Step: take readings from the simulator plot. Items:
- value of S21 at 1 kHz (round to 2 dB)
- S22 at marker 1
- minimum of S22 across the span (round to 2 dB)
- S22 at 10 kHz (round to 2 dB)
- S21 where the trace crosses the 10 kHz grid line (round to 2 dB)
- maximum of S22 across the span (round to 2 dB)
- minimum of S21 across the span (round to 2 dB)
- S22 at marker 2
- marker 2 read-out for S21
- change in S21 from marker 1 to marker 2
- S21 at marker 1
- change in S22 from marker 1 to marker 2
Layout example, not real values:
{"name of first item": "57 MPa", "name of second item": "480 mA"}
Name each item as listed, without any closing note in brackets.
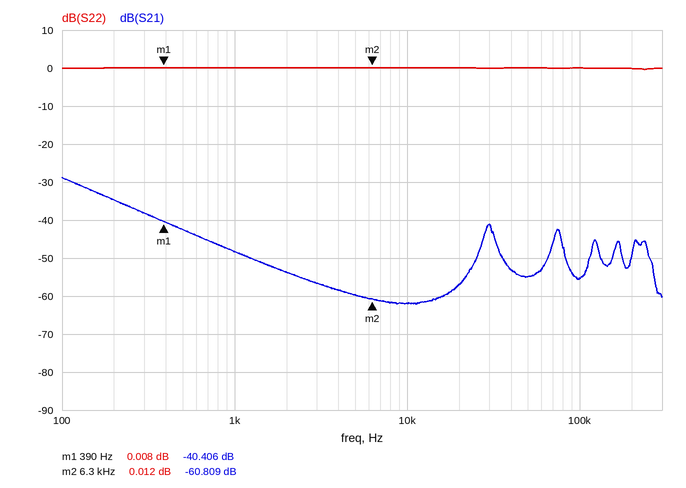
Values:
{"value of S21 at 1 kHz": "-48 dB", "S22 at marker 1": "0.008 dB", "minimum of S22 across the span": "0 dB", "S22 at 10 kHz": "0 dB", "S21 where the trace crosses the 10 kHz grid line": "-62 dB", "maximum of S22 across the span": "0 dB", "minimum of S21 across the span": "-62 dB", "S22 at marker 2": "0.012 dB", "marker 2 read-out for S21": "-60.809 dB", "change in S21 from marker 1 to marker 2": "-20.403 dB", "S21 at marker 1": "-40.406 dB", "change in S22 from marker 1 to marker 2": "0.004 dB"}
